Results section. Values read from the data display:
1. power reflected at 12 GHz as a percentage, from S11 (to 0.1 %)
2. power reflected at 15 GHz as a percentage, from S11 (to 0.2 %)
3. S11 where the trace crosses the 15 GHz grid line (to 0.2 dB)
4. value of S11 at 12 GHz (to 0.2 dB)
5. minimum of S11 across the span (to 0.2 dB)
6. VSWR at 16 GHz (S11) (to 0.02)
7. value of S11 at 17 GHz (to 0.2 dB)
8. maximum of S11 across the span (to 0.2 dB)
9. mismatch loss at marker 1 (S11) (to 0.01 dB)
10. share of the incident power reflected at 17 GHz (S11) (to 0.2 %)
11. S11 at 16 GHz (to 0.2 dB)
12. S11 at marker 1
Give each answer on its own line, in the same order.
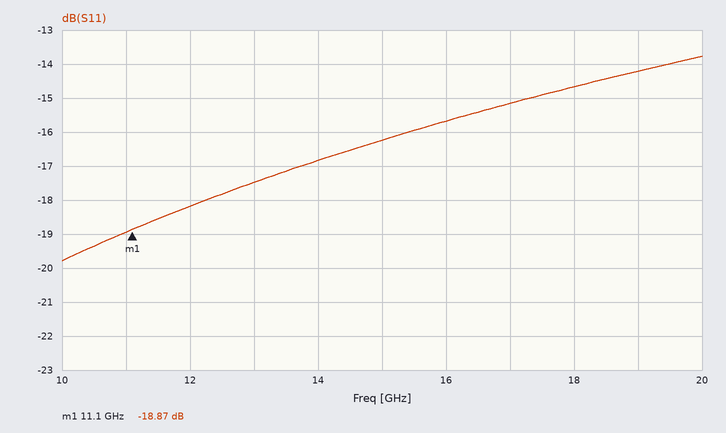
1.5 %
2.4 %
-16.2 dB
-18.2 dB
-19.8 dB
1.40
-15.2 dB
-13.8 dB
0.06 dB
3.0 %
-15.6 dB
-18.87 dB
